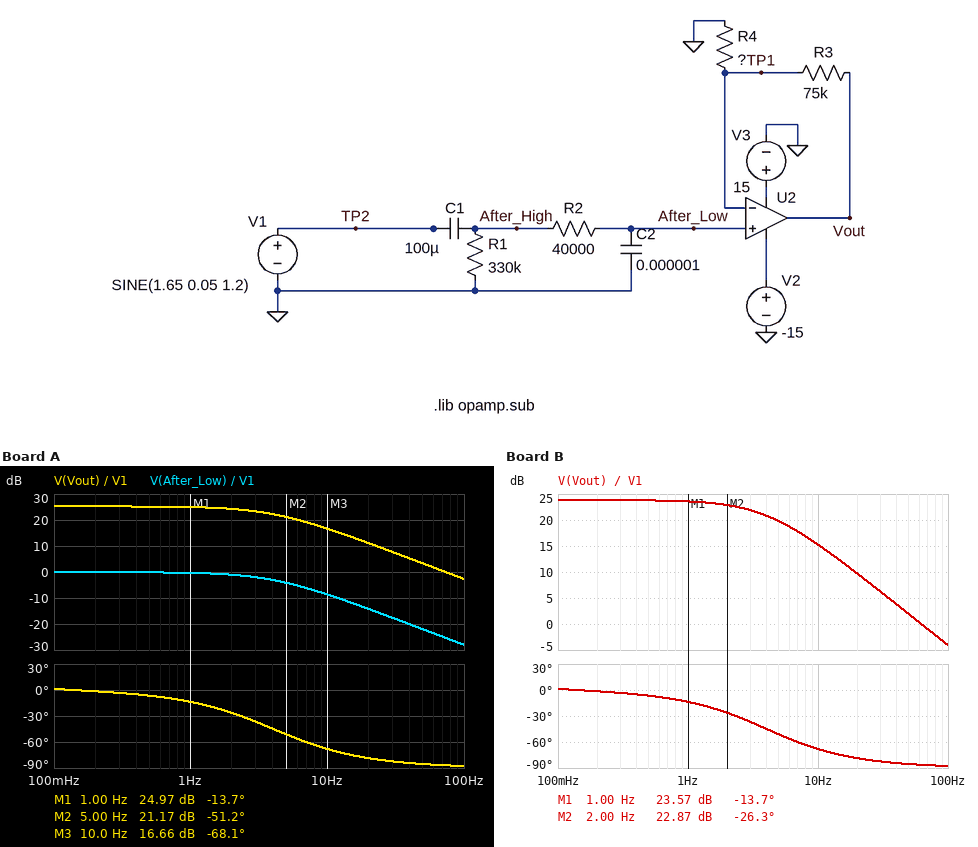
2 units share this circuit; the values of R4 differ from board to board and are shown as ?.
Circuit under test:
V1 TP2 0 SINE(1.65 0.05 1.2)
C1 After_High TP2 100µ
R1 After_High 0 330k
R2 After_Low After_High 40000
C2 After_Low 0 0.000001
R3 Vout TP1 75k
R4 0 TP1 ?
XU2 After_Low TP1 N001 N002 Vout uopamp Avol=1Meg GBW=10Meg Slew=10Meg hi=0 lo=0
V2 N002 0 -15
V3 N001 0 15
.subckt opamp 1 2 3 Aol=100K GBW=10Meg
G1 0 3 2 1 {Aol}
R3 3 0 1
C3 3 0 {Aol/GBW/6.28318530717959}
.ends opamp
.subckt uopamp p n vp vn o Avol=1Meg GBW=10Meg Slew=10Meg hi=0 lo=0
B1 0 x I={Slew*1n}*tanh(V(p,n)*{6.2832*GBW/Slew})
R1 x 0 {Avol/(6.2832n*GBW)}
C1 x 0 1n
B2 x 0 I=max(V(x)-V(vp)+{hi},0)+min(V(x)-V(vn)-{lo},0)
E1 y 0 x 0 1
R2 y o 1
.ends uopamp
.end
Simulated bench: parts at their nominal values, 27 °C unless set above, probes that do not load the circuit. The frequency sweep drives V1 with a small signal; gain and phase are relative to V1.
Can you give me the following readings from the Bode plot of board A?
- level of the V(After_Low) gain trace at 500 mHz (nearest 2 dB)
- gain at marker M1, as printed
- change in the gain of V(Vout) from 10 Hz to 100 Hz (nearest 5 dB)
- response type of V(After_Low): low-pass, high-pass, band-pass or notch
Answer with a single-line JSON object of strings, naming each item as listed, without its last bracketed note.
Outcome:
{"level of the V(After_Low) gain trace at 500 mHz": "0 dB", "gain at marker M1, as printed": "24.97 dB", "change in the gain of V(Vout) from 10 Hz to 100 Hz": "-20 dB", "response type of V(After_Low): low-pass, high-pass, band-pass or notch": "low-pass"}
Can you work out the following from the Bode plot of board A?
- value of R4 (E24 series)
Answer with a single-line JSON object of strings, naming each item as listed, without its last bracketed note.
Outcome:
{"value of R4": "4.3 kΩ"}
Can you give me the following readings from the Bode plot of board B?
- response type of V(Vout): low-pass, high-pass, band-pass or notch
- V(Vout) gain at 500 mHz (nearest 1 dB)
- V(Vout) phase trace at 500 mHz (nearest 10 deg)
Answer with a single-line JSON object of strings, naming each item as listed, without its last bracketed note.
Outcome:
{"response type of V(Vout): low-pass, high-pass, band-pass or notch": "low-pass", "V(Vout) gain at 500 mHz": "24 dB", "V(Vout) phase trace at 500 mHz": "-10 deg"}
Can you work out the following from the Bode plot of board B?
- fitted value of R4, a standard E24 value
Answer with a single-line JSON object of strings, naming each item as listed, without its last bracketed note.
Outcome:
{"fitted value of R4, a standard E24 value": "5.1 kΩ"}
